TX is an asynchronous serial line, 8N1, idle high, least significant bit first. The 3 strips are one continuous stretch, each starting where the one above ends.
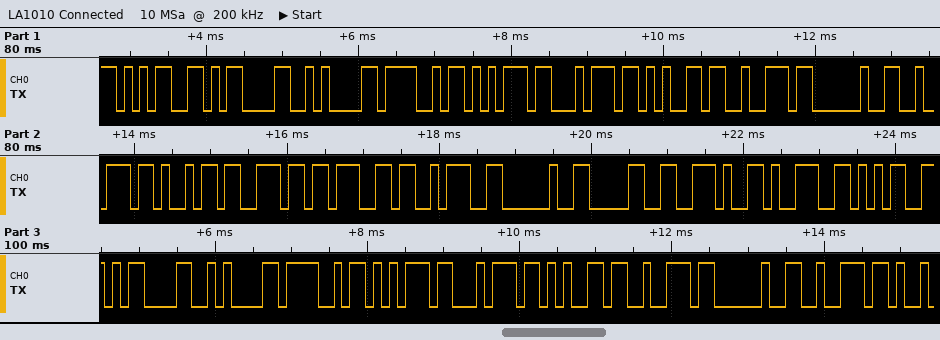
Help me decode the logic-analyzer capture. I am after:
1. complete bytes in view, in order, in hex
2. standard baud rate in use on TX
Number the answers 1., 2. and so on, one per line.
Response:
1. 35 0D 0A 4F 75 74 65 72 20 72 69 6E 67 3A 20 30 2E 39 35 0D 0A 4F 75 74 65 72 20 72
2. 9600 baud
